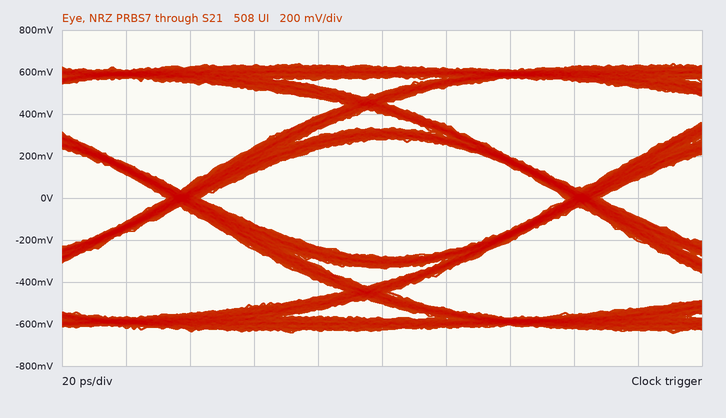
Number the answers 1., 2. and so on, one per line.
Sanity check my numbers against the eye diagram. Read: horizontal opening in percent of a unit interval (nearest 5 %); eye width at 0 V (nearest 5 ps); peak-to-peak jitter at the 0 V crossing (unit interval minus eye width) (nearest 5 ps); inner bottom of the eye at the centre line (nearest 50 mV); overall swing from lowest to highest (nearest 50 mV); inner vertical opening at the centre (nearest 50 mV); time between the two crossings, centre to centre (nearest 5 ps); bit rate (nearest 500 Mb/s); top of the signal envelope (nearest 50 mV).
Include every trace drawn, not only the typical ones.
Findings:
1. 90 %
2. 115 ps
3. 10 ps
4. -300 mV
5. 1.30 V
6. 550 mV
7. 125 ps
8. 8.0 Gb/s
9. 650 mV
